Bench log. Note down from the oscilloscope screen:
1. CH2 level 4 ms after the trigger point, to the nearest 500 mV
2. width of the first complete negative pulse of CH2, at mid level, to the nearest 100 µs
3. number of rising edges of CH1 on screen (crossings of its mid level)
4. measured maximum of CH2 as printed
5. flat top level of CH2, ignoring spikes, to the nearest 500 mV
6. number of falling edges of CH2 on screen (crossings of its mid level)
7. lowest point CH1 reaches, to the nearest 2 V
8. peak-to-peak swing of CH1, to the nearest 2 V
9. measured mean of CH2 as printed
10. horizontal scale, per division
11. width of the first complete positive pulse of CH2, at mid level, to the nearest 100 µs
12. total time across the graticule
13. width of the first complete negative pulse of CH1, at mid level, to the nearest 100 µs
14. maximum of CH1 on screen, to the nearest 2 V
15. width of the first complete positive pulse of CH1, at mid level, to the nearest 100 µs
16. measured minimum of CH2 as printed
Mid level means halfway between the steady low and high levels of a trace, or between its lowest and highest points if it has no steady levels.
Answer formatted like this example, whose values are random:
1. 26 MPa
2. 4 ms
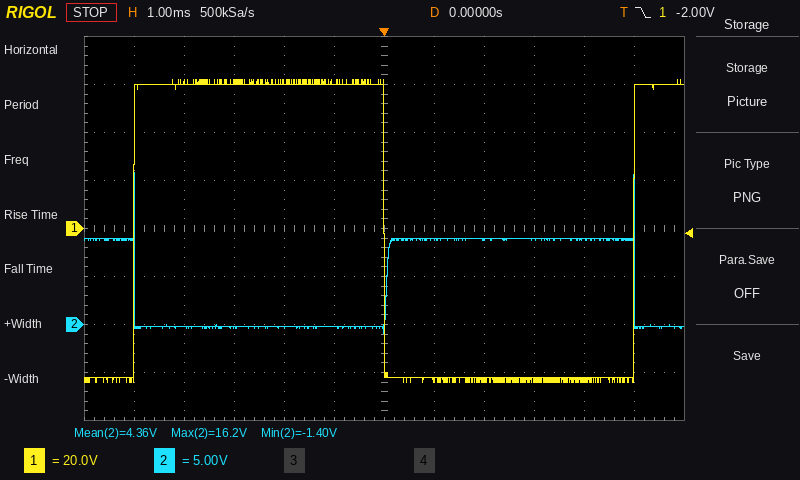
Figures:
1. 9.0 V
2. 5.0 ms
3. 2
4. 16.2 V
5. 9.0 V
6. 2
7. -64 V
8. 126 V
9. 4.36 V
10. 1 ms
11. 5.0 ms
12. 12 ms
13. 5.0 ms
14. 62 V
15. 5.0 ms
16. -1.40 V
